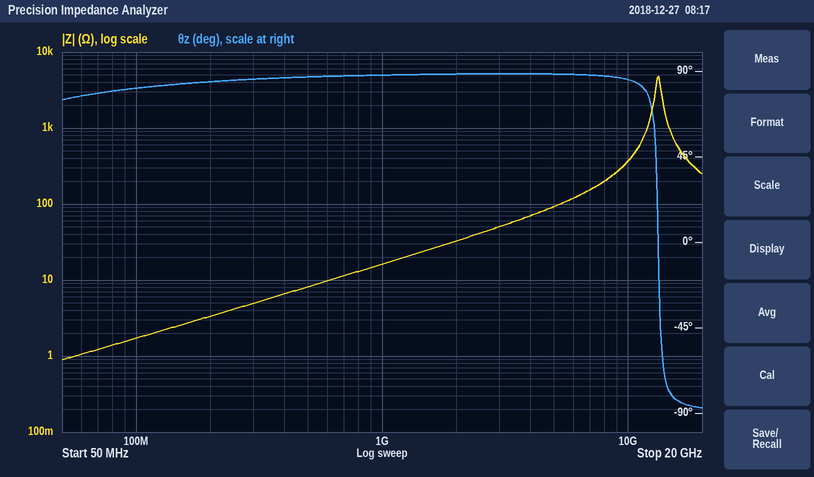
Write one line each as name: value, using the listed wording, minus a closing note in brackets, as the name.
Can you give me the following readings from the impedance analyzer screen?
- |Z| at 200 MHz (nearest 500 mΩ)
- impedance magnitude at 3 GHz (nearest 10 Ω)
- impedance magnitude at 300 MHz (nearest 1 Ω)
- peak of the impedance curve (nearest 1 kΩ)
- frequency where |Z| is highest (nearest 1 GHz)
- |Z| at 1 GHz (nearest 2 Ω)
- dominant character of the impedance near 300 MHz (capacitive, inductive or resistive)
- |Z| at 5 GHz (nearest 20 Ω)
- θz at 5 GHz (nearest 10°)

|Z| at 200 MHz: 3.5 Ω
impedance magnitude at 3 GHz: 50 Ω
impedance magnitude at 300 MHz: 5 Ω
peak of the impedance curve: 5 kΩ
frequency where |Z| is highest: 13 GHz
|Z| at 1 GHz: 16 Ω
dominant character of the impedance near 300 MHz: inductive
|Z| at 5 GHz: 100 Ω
θz at 5 GHz: 90°
